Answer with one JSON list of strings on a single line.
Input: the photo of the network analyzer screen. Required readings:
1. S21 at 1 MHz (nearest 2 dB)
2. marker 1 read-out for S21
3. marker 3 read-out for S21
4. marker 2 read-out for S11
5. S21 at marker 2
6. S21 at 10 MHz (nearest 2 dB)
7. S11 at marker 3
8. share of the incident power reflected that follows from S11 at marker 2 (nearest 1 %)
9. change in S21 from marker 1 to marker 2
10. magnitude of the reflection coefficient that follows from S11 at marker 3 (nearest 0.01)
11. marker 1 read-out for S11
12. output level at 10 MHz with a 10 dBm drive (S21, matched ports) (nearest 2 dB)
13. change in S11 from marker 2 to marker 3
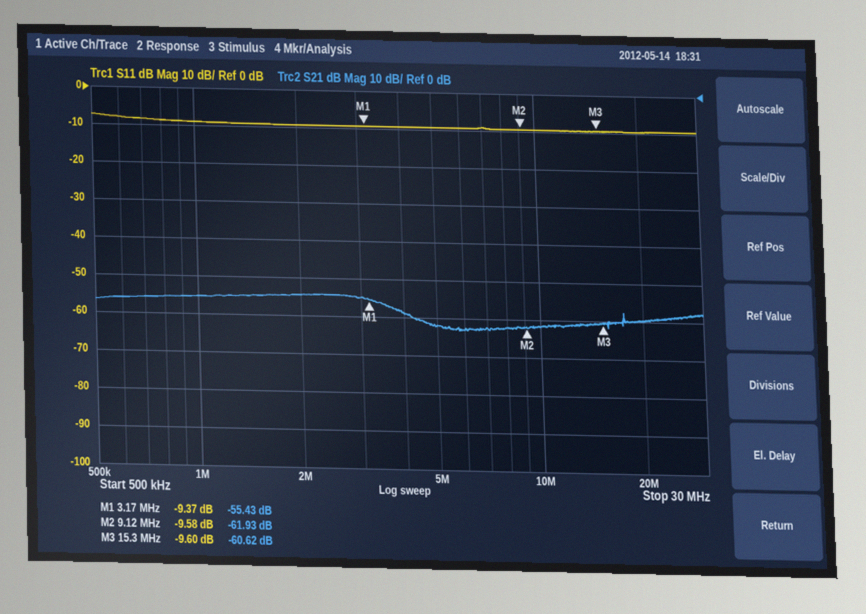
["-56 dB", "-55.43 dB", "-60.62 dB", "-9.58 dB", "-61.93 dB", "-62 dB", "-9.60 dB", "11 %", "-6.50 dB", "0.33", "-9.37 dB", "-52 dBm", "-0.02 dB"]
